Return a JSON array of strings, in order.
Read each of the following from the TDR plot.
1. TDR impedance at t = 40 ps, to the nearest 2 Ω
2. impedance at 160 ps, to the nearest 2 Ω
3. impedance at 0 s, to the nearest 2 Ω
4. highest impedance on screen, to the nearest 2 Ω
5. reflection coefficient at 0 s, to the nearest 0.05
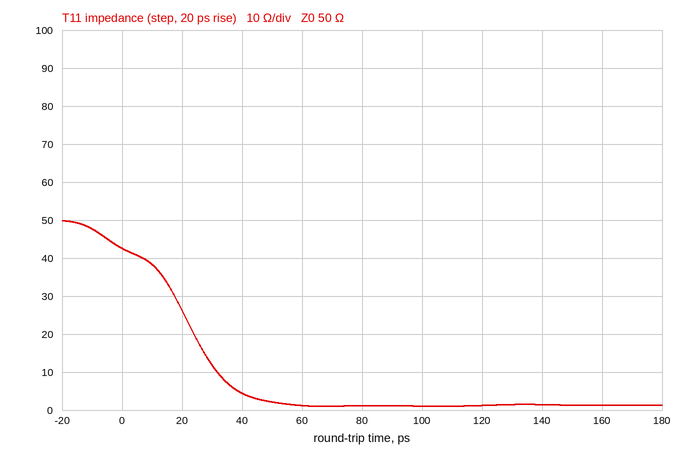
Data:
["4 Ω", "2 Ω", "42 Ω", "50 Ω", "-0.10"]
